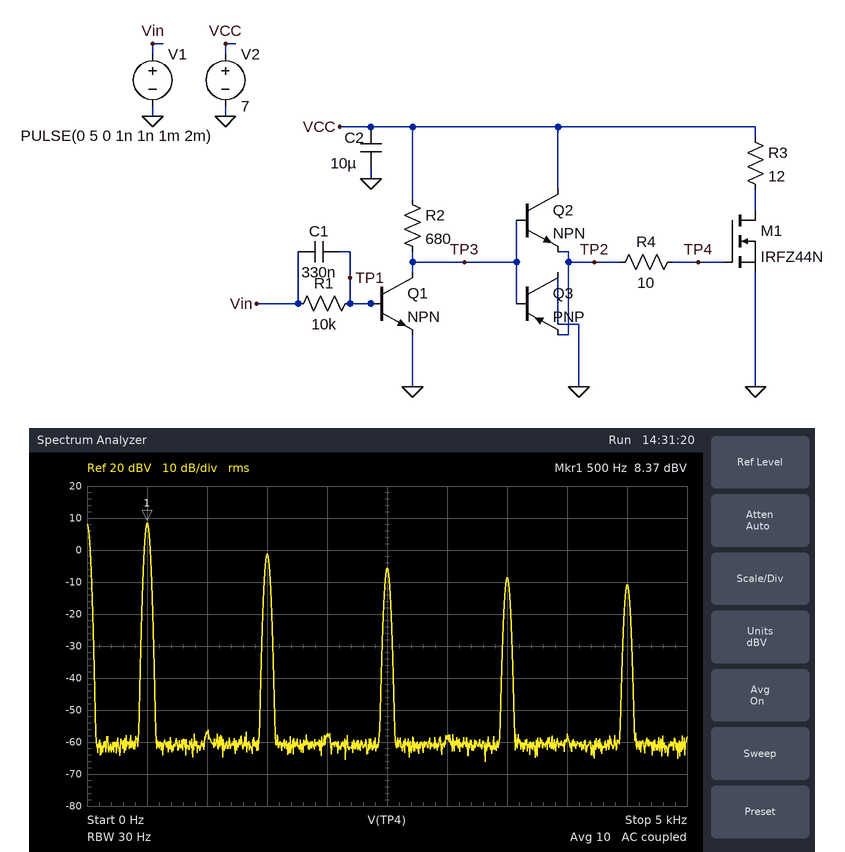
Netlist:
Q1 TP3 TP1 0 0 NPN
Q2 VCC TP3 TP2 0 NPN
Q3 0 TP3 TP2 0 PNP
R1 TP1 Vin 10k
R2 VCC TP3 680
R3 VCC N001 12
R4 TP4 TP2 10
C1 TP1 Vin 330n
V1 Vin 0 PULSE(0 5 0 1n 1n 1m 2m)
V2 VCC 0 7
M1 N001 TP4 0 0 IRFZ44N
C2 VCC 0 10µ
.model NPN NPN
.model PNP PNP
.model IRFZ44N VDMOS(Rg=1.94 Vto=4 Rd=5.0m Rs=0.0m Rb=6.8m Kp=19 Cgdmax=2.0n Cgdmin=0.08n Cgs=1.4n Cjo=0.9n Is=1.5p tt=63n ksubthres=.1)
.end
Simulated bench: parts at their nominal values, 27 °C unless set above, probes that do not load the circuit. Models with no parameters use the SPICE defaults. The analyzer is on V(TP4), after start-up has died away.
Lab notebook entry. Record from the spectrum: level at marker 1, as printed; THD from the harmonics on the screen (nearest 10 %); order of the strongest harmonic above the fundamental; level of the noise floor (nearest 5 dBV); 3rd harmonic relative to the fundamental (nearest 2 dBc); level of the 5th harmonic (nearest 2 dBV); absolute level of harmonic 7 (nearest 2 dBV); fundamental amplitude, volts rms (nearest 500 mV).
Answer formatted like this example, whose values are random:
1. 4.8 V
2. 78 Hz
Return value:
1. 8.37 dBV
2. 40 %
3. 3
4. -60 dBV
5. -10 dBc
6. -6 dBV
7. -8 dBV
8. 2.5 V
